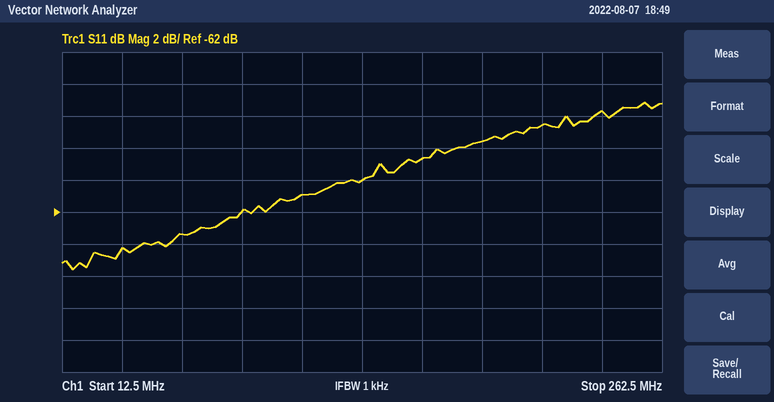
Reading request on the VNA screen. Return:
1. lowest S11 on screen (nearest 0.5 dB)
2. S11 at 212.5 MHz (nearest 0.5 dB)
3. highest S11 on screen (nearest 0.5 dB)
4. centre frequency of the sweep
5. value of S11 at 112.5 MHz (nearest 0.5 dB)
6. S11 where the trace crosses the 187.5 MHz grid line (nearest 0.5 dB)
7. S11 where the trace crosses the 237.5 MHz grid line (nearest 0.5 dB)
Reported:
-65.5 dB
-56.5 dB
-55.0 dB
137.5 MHz
-61.0 dB
-57.5 dB
-55.5 dB
